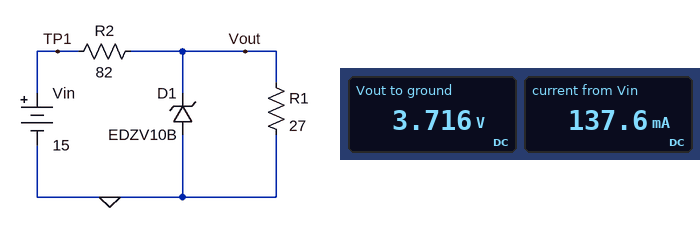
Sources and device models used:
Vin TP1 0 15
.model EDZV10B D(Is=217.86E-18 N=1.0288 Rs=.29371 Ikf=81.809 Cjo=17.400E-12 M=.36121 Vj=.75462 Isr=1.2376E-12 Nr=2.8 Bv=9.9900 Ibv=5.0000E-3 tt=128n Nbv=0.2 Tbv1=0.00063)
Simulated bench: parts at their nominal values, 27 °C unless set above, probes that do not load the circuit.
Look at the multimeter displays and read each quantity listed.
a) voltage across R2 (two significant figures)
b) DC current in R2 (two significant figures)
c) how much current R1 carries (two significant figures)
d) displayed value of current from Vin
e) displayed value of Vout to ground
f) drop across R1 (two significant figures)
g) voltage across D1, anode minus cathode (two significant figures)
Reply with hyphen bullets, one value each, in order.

- 11 V
- 140 mA
- 140 mA
- 137.6 mA
- 3.716 V
- 3.7 V
- -3.7 V
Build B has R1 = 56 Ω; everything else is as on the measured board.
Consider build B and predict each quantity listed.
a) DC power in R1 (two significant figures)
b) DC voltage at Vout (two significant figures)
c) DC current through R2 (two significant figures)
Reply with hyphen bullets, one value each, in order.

- 660 mW
- 6.1 V
- 110 mA
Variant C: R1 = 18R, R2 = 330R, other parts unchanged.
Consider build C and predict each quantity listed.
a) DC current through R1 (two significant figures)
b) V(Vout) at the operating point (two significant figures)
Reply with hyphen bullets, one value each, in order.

- 43 mA
- 780 mV
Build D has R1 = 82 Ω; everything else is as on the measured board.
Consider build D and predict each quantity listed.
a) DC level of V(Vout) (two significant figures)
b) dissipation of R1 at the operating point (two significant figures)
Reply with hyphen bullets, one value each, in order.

- 7.5 V
- 690 mW
